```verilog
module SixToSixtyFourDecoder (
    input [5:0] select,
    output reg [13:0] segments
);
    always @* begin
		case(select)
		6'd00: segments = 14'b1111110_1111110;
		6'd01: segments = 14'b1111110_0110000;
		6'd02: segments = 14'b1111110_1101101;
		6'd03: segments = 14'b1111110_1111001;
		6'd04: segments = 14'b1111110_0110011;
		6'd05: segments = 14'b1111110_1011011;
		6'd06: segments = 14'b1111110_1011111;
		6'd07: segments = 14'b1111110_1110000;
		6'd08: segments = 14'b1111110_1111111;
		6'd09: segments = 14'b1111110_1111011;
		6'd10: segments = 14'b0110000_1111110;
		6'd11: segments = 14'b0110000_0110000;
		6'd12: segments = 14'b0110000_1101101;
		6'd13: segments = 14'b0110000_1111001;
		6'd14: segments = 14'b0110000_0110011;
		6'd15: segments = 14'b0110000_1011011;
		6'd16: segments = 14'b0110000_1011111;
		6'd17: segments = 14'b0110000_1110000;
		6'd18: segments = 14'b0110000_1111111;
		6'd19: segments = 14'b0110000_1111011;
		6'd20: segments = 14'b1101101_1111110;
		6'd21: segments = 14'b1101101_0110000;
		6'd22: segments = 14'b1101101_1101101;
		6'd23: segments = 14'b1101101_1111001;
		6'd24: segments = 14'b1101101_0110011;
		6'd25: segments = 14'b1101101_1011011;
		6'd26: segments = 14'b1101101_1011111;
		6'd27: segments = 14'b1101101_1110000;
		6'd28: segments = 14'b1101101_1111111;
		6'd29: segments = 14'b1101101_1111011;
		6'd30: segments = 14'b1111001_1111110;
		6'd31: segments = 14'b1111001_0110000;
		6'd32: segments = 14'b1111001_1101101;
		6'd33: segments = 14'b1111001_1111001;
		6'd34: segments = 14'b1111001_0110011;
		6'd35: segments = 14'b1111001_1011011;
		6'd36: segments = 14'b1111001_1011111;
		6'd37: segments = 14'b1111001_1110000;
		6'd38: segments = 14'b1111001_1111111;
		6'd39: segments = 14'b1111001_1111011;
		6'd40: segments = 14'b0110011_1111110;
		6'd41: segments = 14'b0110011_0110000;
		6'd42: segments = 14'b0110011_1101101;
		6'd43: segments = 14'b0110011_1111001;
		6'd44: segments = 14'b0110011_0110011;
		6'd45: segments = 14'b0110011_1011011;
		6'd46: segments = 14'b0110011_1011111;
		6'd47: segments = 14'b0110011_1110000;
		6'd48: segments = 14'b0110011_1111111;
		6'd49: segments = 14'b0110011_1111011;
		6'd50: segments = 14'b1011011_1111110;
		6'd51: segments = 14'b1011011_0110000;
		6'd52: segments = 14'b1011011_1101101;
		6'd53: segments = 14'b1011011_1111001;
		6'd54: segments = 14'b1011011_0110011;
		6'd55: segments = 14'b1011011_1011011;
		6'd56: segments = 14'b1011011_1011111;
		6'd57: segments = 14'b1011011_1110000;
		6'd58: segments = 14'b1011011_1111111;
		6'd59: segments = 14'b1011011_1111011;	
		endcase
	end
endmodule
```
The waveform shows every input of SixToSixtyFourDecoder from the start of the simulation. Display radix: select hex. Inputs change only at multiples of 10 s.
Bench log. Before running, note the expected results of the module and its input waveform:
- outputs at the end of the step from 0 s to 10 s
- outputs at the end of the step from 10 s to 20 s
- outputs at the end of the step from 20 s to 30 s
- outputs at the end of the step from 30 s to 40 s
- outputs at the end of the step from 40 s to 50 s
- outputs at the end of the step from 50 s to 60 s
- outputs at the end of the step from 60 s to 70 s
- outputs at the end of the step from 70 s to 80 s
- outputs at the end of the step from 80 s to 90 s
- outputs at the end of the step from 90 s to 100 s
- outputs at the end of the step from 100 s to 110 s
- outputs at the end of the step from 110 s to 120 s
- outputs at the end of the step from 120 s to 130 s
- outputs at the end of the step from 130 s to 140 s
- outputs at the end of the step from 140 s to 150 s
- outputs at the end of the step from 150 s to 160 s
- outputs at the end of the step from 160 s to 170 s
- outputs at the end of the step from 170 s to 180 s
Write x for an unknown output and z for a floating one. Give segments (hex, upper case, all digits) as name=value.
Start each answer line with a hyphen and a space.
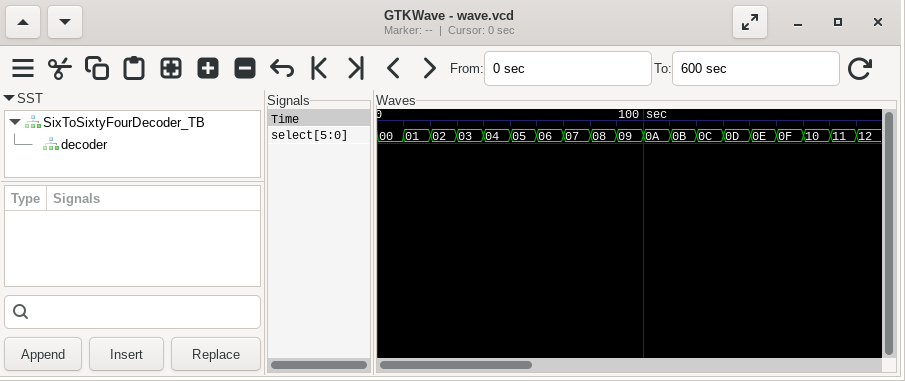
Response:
- segments=3F7E
- segments=3F30
- segments=3F6D
- segments=3F79
- segments=3F33
- segments=3F5B
- segments=3F5F
- segments=3F70
- segments=3F7F
- segments=3F7B
- segments=187E
- segments=1830
- segments=186D
- segments=1879
- segments=1833
- segments=185B
- segments=185F
- segments=1870
